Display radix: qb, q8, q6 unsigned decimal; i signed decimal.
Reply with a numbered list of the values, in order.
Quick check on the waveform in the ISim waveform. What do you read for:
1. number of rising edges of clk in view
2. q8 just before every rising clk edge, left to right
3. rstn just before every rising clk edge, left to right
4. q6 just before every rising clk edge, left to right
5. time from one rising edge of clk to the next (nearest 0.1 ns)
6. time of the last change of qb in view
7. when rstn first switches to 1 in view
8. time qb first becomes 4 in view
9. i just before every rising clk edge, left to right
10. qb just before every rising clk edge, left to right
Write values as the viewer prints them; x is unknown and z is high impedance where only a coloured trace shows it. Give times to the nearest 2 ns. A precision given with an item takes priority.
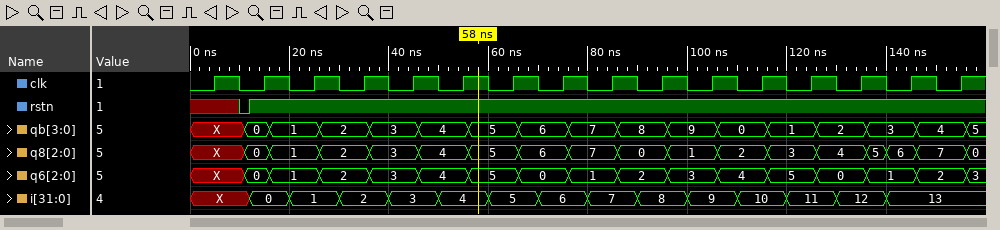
1. 16
2. X, 0, 1, 2, 3, 4, 5, 6, 7, 0, 1, 2, 3, 4, 6, 7
3. x 1 1 1 1 1 1 1 1 1 1 1 1 1 1 1
4. X, 0, 1, 2, 3, 4, 5, 0, 1, 2, 3, 4, 5, 0, 1, 2
5. 10 ns
6. 156 ns
7. 12 ns
8. 46 ns
9. X, 0, 1, 2, 3, 4, 5, 6, 7, 8, 9, 10, 11, 12, 13, 13
10. X, 0, 1, 2, 3, 4, 5, 6, 7, 8, 9, 0, 1, 2, 3, 4
